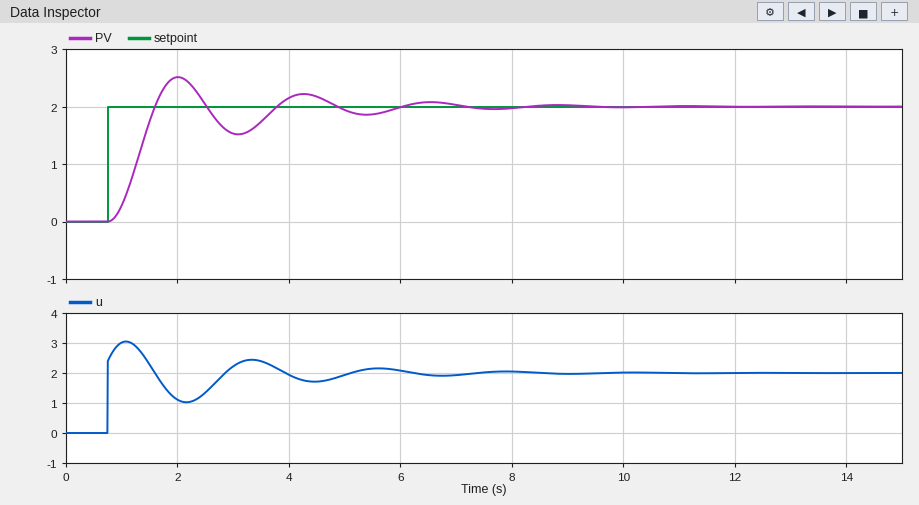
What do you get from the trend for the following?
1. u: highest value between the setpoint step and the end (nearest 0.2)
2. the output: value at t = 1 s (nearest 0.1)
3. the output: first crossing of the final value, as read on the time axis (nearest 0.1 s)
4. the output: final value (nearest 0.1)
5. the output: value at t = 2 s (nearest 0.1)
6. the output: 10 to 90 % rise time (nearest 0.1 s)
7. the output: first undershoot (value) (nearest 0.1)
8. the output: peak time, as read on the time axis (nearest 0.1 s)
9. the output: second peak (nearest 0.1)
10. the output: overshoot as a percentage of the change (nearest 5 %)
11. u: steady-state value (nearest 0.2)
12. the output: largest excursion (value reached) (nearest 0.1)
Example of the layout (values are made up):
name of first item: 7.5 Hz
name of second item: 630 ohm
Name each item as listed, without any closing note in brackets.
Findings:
u: highest value between the setpoint step and the end: 3.0
the output: value at t = 1 s: 0.3
the output: first crossing of the final value, as read on the time axis: 1.6 s
the output: final value: 2.0
the output: value at t = 2 s: 2.5
the output: 10 to 90 % rise time: 0.6 s
the output: first undershoot (value): 1.5
the output: peak time, as read on the time axis: 2.0 s
the output: second peak: 2.2
the output: overshoot as a percentage of the change: 25 %
u: steady-state value: 2.0
the output: largest excursion (value reached): 2.5
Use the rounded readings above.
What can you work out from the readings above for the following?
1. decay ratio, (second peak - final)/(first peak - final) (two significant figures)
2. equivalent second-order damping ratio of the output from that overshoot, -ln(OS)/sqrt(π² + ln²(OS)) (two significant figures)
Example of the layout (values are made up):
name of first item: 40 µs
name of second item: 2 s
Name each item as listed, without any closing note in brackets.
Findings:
decay ratio, (second peak - final)/(first peak - final): 0.40
equivalent second-order damping ratio of the output from that overshoot, -ln(OS)/sqrt(π² + ln²(OS)): 0.40
